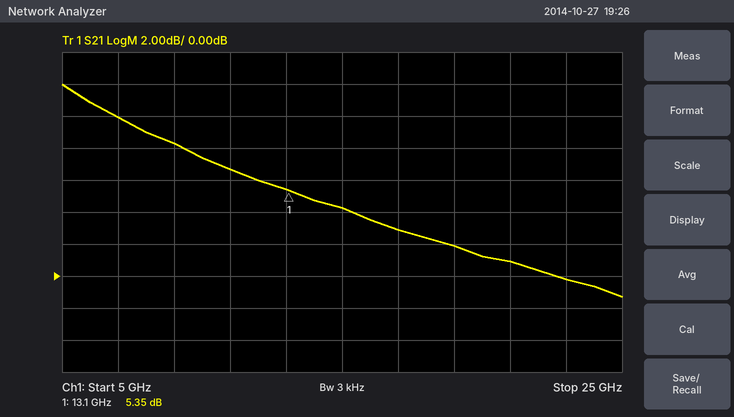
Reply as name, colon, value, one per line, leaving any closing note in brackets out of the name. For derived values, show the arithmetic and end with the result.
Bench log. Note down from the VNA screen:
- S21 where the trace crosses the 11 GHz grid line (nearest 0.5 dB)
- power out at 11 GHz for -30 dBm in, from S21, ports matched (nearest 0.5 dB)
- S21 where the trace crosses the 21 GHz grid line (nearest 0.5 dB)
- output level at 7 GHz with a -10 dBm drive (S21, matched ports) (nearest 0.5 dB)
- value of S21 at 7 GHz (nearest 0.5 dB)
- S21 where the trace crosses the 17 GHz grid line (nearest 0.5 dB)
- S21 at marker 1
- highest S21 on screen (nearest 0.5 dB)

S21 where the trace crosses the 11 GHz grid line: 6.5 dB
power out at 11 GHz for -30 dBm in, from S21, ports matched: -30 dBm + (6.5 dB) = -23.5 dBm
S21 where the trace crosses the 21 GHz grid line: 1.0 dB
output level at 7 GHz with a -10 dBm drive (S21, matched ports): -10 dBm + (10.0 dB) = 0.0 dBm
value of S21 at 7 GHz: 10.0 dB
S21 where the trace crosses the 17 GHz grid line: 3.0 dB
S21 at marker 1: 5.35 dB
highest S21 on screen: 12.0 dB
